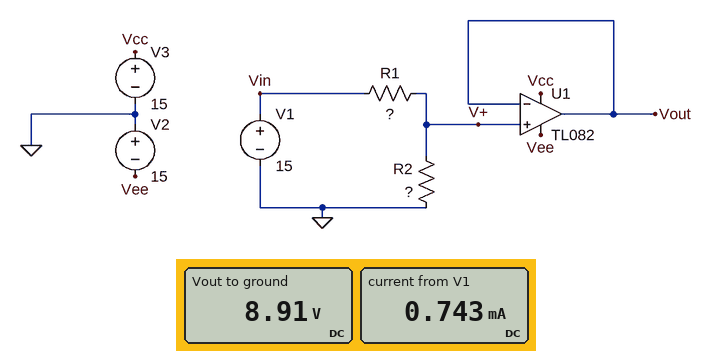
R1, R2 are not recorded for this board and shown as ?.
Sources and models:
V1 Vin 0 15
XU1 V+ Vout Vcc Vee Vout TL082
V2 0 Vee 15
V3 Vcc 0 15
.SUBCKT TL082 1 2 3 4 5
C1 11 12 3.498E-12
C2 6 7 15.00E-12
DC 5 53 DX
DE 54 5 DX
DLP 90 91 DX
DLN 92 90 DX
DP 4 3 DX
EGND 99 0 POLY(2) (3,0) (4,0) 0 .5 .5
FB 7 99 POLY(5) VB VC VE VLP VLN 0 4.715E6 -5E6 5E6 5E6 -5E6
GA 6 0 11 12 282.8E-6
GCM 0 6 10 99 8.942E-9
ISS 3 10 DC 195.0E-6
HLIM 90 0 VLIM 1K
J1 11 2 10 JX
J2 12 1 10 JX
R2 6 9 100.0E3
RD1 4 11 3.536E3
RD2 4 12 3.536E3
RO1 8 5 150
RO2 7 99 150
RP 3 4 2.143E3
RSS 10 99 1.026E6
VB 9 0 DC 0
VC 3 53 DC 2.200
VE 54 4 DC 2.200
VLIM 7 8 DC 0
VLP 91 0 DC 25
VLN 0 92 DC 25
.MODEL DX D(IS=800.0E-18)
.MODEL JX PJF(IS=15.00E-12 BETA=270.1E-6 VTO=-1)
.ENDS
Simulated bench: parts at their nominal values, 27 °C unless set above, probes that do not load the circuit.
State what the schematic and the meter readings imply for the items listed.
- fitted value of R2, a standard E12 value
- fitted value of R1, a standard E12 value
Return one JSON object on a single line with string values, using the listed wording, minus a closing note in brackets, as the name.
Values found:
{"fitted value of R2, a standard E12 value": "12 kΩ", "fitted value of R1, a standard E12 value": "8.2 kΩ"}
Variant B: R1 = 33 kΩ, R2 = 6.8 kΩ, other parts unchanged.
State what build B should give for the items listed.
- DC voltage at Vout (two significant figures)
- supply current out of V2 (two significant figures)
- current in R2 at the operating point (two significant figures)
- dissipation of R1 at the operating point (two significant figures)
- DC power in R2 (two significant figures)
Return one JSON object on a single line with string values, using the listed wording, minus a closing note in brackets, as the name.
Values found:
{"DC voltage at Vout": "2.6 V", "supply current out of V2": "14 mA", "current in R2 at the operating point": "380 µA", "dissipation of R1 at the operating point": "4.7 mW", "DC power in R2": "970 µW"}
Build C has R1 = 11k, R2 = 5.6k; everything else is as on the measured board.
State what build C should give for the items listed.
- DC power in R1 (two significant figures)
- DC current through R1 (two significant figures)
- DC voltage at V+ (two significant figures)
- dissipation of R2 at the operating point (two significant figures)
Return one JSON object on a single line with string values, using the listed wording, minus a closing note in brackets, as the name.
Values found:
{"DC power in R1": "9.0 mW", "DC current through R1": "900 µA", "DC voltage at V+": "5.1 V", "dissipation of R2 at the operating point": "4.6 mW"}
